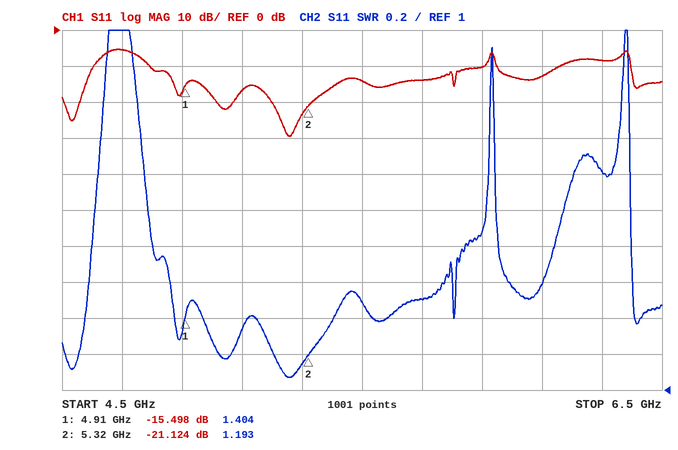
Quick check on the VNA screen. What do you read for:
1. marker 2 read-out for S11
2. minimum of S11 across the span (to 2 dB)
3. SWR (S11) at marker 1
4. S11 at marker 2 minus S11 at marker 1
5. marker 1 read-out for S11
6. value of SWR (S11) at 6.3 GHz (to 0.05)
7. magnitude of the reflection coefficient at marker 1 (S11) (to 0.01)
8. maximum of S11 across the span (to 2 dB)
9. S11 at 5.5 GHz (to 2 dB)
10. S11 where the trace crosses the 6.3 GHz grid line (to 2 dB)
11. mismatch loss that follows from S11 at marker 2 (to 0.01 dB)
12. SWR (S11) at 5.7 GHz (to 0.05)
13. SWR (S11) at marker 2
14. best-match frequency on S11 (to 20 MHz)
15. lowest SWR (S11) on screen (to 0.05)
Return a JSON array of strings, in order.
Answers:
["-21.124 dB", "-30 dB", "1.404", "-5.626 dB", "-15.498 dB", "2.20", "0.17", "-6 dB", "-14 dB", "-8 dB", "0.03 dB", "1.50", "1.193", "5.26 GHz", "1.05"]
